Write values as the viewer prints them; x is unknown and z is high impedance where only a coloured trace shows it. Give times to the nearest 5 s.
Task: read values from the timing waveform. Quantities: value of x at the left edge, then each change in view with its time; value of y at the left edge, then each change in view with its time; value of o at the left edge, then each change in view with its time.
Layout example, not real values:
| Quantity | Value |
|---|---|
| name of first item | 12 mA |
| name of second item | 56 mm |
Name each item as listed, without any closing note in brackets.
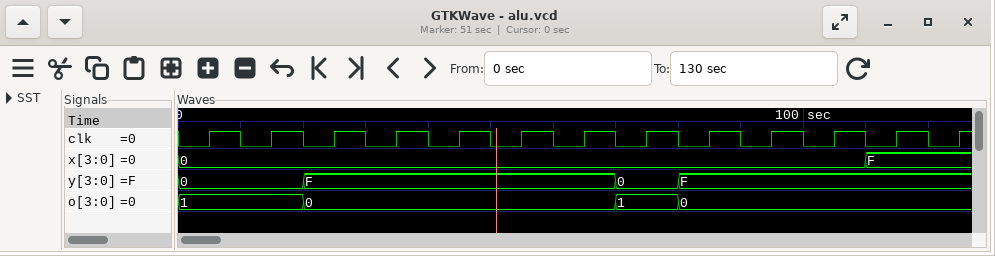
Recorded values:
| Quantity | Value |
|---|---|
| value of x at the left edge, then each change in view with its time | 0, F at 110 s |
| value of y at the left edge, then each change in view with its time | 0, F at 20 s, 0 at 70 s, F at 80 s |
| value of o at the left edge, then each change in view with its time | 1, 0 at 20 s, 1 at 70 s, 0 at 80 s |
